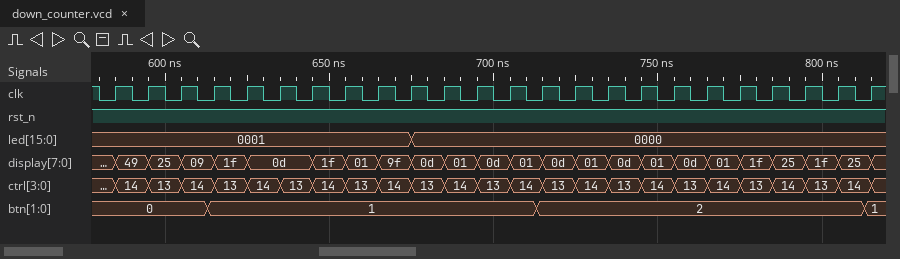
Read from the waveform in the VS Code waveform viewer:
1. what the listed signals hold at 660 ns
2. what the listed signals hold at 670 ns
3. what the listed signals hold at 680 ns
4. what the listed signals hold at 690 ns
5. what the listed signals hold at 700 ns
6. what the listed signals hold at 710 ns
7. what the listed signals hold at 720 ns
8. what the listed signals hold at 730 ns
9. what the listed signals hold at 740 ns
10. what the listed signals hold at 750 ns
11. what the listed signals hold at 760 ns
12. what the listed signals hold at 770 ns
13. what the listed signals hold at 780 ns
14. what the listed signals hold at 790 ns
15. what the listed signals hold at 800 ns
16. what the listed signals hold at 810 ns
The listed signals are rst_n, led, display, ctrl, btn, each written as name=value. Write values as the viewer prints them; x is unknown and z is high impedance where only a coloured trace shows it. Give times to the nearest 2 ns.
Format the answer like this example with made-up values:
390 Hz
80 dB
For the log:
rst_n=1, led=0001, display=01, ctrl=13, btn=1
rst_n=1, led=0001, display=9f, ctrl=14, btn=1
rst_n=1, led=0000, display=0d, ctrl=13, btn=1
rst_n=1, led=0000, display=01, ctrl=14, btn=1
rst_n=1, led=0000, display=0d, ctrl=13, btn=1
rst_n=1, led=0000, display=01, ctrl=14, btn=1
rst_n=1, led=0000, display=0d, ctrl=13, btn=2
rst_n=1, led=0000, display=01, ctrl=14, btn=2
rst_n=1, led=0000, display=0d, ctrl=13, btn=2
rst_n=1, led=0000, display=01, ctrl=14, btn=2
rst_n=1, led=0000, display=0d, ctrl=13, btn=2
rst_n=1, led=0000, display=01, ctrl=14, btn=2
rst_n=1, led=0000, display=1f, ctrl=13, btn=2
rst_n=1, led=0000, display=25, ctrl=14, btn=2
rst_n=1, led=0000, display=1f, ctrl=13, btn=2
rst_n=1, led=0000, display=25, ctrl=14, btn=2
